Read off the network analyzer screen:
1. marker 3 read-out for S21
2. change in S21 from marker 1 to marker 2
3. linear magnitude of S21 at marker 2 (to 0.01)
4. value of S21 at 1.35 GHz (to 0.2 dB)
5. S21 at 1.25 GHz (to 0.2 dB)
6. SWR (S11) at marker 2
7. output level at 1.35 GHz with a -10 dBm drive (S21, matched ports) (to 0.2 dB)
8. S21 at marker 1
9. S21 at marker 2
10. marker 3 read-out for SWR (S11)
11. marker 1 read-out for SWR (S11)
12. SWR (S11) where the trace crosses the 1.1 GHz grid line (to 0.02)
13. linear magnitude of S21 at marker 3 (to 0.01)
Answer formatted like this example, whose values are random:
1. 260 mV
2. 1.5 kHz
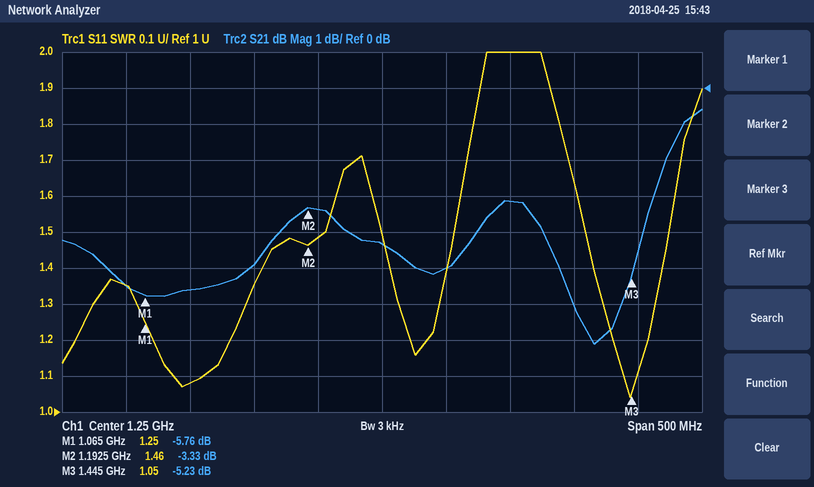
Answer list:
1. -5.23 dB
2. 2.43 dB
3. 0.68
4. -3.2 dB
5. -4.4 dB
6. 1.46
7. -13.2 dBm
8. -5.76 dB
9. -3.33 dB
10. 1.05
11. 1.25
12. 1.08
13. 0.55
